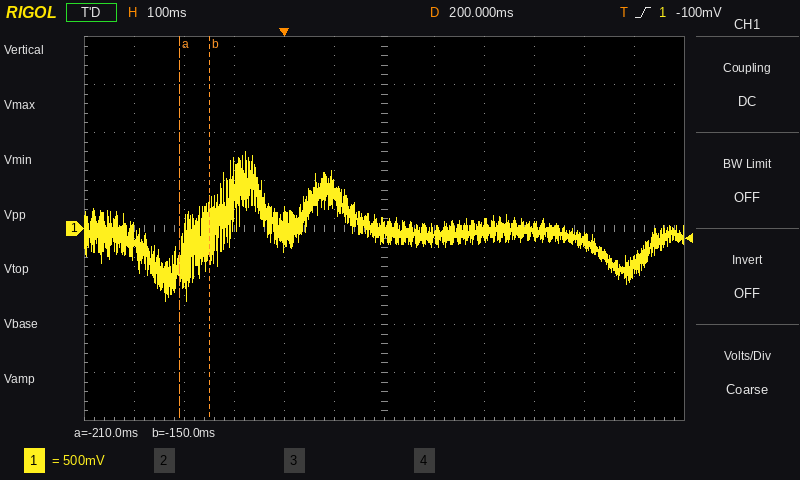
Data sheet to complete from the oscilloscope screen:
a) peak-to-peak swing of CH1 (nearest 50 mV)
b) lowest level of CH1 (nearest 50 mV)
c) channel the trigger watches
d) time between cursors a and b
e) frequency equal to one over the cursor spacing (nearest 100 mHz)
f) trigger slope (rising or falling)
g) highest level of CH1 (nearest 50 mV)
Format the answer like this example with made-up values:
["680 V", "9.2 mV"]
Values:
["1.55 V", "-750 mV", "CH1", "60 ms", "16.7 Hz", "rising", "800 mV"]
